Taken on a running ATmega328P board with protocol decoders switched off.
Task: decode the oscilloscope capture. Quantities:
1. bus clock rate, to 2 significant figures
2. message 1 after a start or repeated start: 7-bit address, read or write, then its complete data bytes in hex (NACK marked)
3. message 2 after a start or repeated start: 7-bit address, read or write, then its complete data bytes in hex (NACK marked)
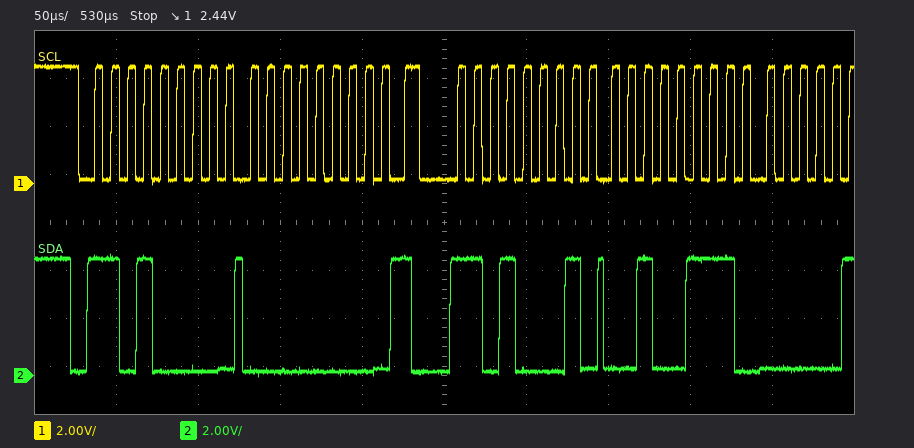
100 kHz
0x68 write: 00
0x68 read: 27
